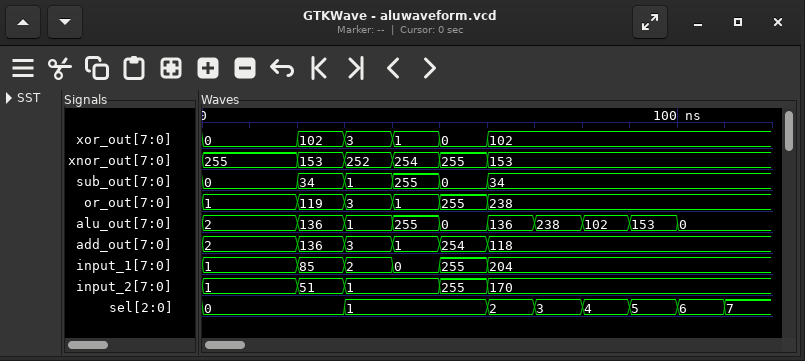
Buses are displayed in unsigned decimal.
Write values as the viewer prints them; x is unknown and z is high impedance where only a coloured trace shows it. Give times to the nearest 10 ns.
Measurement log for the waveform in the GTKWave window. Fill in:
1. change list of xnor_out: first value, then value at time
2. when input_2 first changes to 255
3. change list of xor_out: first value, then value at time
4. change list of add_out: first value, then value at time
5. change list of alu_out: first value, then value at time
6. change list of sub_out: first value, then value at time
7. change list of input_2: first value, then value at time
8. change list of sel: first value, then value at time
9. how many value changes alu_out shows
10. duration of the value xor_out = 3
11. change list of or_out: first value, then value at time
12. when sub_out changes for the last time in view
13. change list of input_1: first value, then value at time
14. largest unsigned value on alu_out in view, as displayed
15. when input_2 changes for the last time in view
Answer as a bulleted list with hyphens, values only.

- 255, 153 at 20 ns, 252 at 30 ns, 254 at 40 ns, 255 at 50 ns, 153 at 60 ns
- 50 ns
- 0, 102 at 20 ns, 3 at 30 ns, 1 at 40 ns, 0 at 50 ns, 102 at 60 ns
- 2, 136 at 20 ns, 3 at 30 ns, 1 at 40 ns, 254 at 50 ns, 118 at 60 ns
- 2, 136 at 20 ns, 1 at 30 ns, 255 at 40 ns, 0 at 50 ns, 136 at 60 ns, 238 at 70 ns, 102 at 80 ns, 153 at 90 ns, 0 at 100 ns
- 0, 34 at 20 ns, 1 at 30 ns, 255 at 40 ns, 0 at 50 ns, 34 at 60 ns
- 1, 51 at 20 ns, 1 at 30 ns, 255 at 50 ns, 170 at 60 ns
- 0, 1 at 30 ns, 2 at 60 ns, 3 at 70 ns, 4 at 80 ns, 5 at 90 ns, 6 at 100 ns, 7 at 110 ns
- 9
- 10 ns
- 1, 119 at 20 ns, 3 at 30 ns, 1 at 40 ns, 255 at 50 ns, 238 at 60 ns
- 60 ns
- 1, 85 at 20 ns, 2 at 30 ns, 0 at 40 ns, 255 at 50 ns, 204 at 60 ns
- 255
- 60 ns
